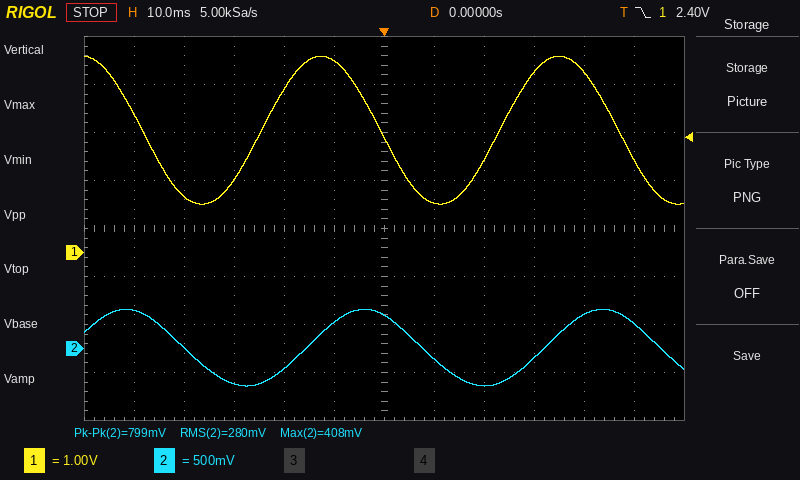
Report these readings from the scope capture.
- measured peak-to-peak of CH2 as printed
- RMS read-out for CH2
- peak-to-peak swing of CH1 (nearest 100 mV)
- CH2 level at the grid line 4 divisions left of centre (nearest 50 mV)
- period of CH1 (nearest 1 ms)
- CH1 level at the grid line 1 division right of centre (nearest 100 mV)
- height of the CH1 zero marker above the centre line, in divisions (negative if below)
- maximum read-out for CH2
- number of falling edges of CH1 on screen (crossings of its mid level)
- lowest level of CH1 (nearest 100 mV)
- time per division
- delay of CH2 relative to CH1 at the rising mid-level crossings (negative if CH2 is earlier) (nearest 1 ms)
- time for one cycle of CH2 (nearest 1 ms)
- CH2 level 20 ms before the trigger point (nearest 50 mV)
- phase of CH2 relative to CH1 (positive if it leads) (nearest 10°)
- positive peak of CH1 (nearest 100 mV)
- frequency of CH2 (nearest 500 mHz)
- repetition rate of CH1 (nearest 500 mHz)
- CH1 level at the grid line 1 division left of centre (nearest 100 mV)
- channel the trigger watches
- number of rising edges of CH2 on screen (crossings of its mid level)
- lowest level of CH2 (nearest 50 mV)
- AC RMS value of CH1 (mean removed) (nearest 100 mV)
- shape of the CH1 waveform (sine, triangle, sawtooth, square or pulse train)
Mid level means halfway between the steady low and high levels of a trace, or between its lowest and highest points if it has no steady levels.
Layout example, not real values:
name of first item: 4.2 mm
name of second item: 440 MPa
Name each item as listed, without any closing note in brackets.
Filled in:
measured peak-to-peak of CH2 as printed: 799 mV
RMS read-out for CH2: 280 mV
peak-to-peak swing of CH1: 3.1 V
CH2 level at the grid line 4 divisions left of centre: 0 mV
period of CH1: 48 ms
CH1 level at the grid line 1 division right of centre: 1.0 V
height of the CH1 zero marker above the centre line, in divisions: -0.5 div
maximum read-out for CH2: 408 mV
number of falling edges of CH1 on screen: 3
lowest level of CH1: 1.0 V
time per division: 10 ms
delay of CH2 relative to CH1 at the rising mid-level crossings (negative if CH2 is earlier): +9 ms
time for one cycle of CH2: 48 ms
CH2 level 20 ms before the trigger point: -200 mV
phase of CH2 relative to CH1 (positive if it leads): -70°
positive peak of CH1: 4.1 V
frequency of CH2: 21.0 Hz
repetition rate of CH1: 21.0 Hz
CH1 level at the grid line 1 division left of centre: 4.0 V
channel the trigger watches: CH1
number of rising edges of CH2 on screen: 2
lowest level of CH2: -400 mV
AC RMS value of CH1 (mean removed): 1.1 V
shape of the CH1 waveform: sine
